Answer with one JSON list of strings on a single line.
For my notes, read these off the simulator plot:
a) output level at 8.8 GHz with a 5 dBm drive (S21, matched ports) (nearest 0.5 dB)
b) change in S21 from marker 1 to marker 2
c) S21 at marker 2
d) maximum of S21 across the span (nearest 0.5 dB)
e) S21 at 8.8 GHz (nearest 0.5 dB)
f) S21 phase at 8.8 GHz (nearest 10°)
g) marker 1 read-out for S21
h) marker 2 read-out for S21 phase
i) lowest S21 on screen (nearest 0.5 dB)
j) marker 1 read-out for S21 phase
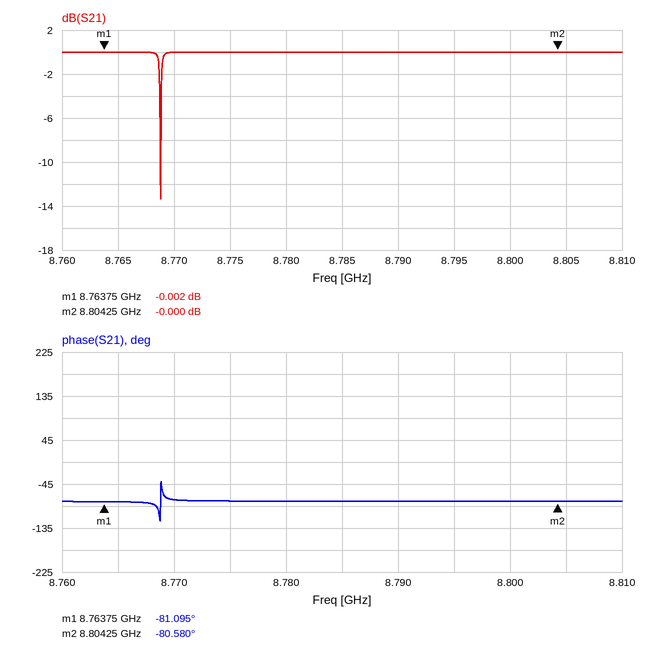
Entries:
["5.0 dBm", "0.002 dB", "-0.000 dB", "0.0 dB", "0.0 dB", "-80°", "-0.002 dB", "-80.580°", "-13.5 dB", "-81.095°"]
